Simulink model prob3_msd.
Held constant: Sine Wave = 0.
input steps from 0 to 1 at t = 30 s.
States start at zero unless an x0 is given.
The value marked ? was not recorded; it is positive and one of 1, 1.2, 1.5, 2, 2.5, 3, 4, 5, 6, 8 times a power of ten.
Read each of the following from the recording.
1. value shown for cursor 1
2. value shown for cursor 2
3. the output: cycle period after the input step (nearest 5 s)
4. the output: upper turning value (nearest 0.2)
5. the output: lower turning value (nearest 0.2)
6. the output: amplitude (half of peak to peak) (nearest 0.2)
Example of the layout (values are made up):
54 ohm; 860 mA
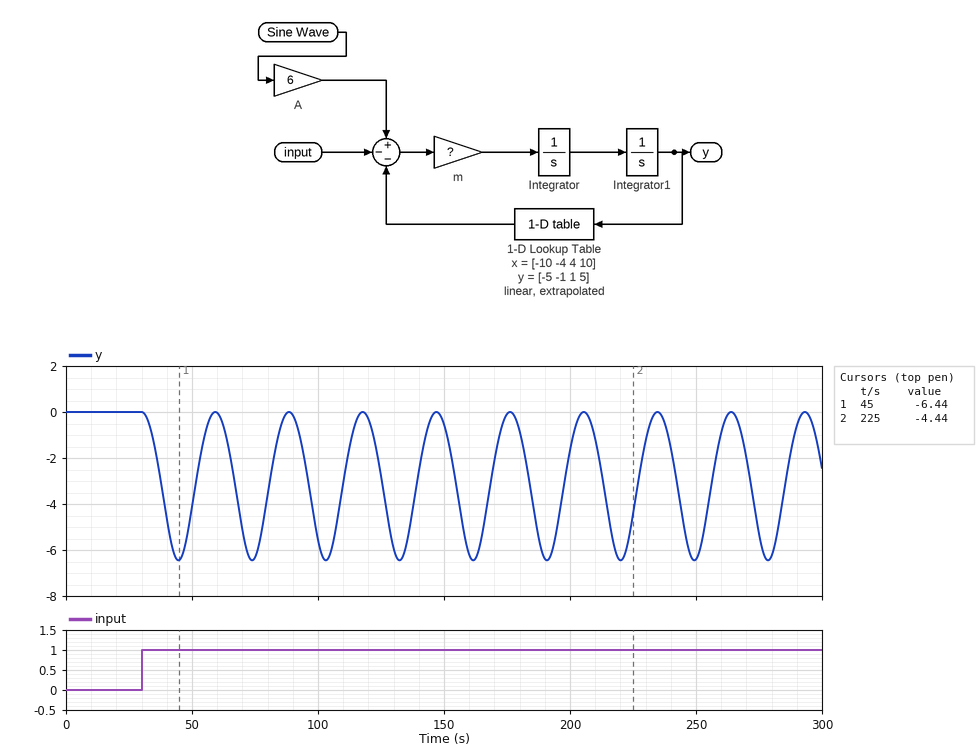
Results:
-6.44; -4.44; 30 s; 0.0; -6.4; 3.2
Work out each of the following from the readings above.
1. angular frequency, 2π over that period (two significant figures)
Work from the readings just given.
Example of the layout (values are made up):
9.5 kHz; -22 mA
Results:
0.21 rad/s
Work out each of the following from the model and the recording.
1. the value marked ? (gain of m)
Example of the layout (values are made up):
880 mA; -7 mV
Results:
0.12
